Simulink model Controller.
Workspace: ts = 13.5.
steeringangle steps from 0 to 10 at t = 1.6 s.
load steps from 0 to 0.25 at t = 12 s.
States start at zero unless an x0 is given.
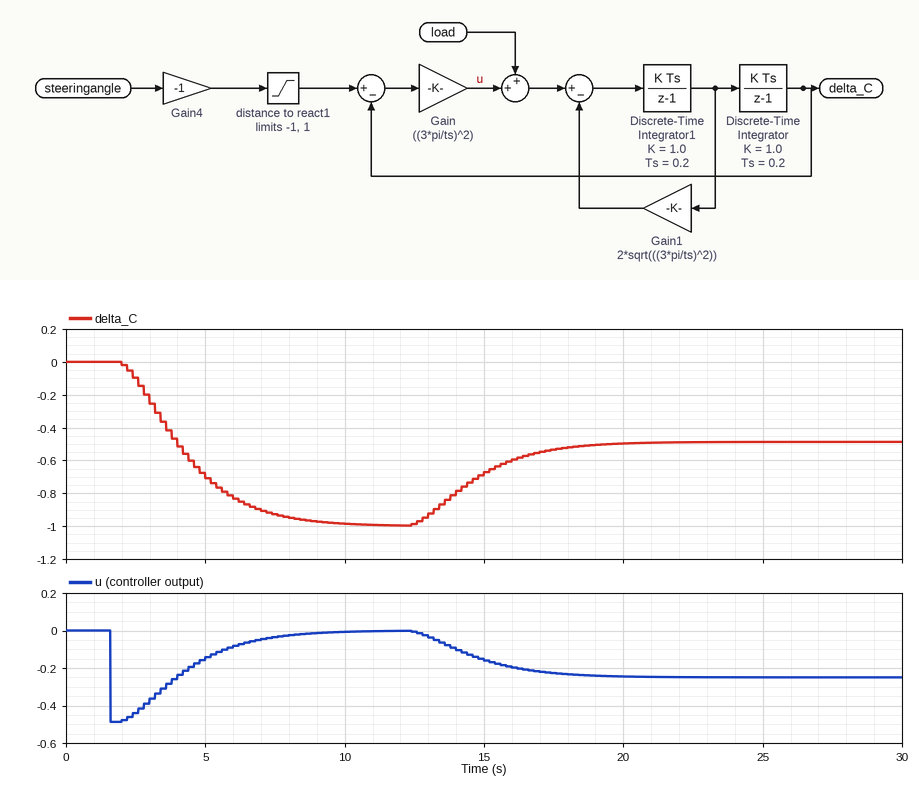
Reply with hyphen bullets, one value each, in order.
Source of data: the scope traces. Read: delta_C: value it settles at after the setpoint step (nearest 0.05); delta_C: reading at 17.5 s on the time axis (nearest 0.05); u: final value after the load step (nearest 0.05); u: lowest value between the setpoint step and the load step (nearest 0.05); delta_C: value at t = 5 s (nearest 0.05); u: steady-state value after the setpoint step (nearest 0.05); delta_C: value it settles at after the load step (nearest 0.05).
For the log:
- -1.00
- -0.55
- -0.25
- -0.50
- -0.70
- 0.00
- -0.50
